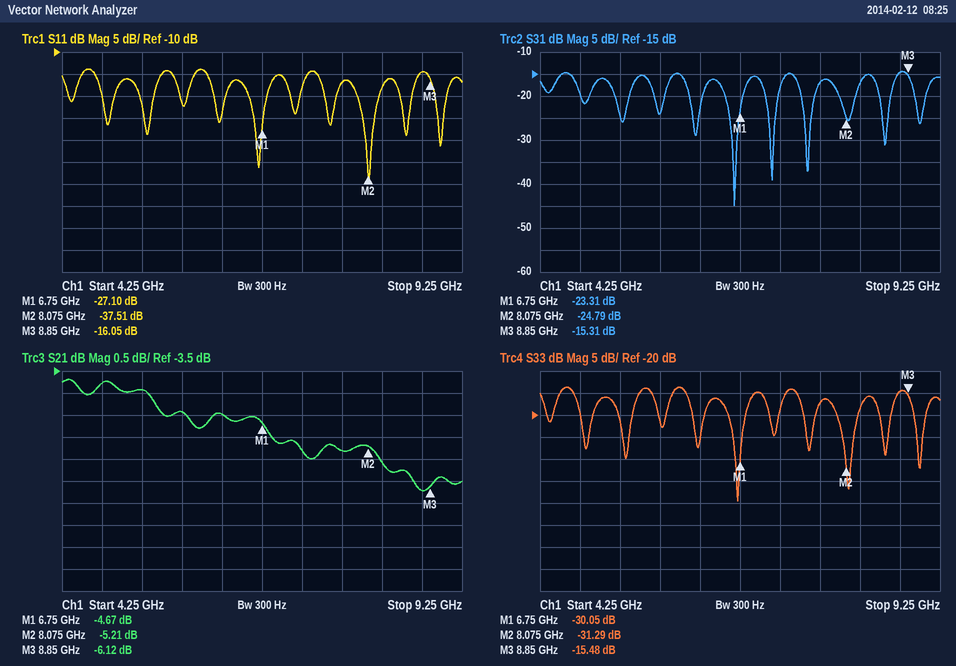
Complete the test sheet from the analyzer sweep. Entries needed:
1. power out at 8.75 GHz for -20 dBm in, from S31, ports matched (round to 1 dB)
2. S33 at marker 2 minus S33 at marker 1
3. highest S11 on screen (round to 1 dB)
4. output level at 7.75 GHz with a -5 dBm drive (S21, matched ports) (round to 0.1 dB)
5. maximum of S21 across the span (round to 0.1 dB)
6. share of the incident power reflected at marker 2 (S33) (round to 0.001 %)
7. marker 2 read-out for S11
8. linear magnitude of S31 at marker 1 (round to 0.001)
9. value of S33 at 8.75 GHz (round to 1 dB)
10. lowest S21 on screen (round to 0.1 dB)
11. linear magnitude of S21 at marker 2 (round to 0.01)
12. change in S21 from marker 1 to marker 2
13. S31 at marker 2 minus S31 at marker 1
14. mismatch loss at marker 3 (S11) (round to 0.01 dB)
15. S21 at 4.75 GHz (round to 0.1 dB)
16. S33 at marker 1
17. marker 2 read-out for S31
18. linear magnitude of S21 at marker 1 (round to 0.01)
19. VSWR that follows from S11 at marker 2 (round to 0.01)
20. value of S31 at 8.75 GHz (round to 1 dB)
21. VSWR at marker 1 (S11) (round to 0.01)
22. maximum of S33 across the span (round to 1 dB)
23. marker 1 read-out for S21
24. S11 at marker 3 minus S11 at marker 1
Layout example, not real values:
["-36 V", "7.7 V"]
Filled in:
["-35 dBm", "-1.24 dB", "-14 dB", "-10.3 dBm", "-3.7 dB", "0.074 %", "-37.51 dB", "0.068", "-15 dB", "-6.2 dB", "0.55", "-0.54 dB", "-1.48 dB", "0.11 dB", "-3.8 dB", "-30.05 dB", "-24.79 dB", "0.58", "1.03", "-15 dB", "1.09", "-14 dB", "-4.67 dB", "11.05 dB"]
